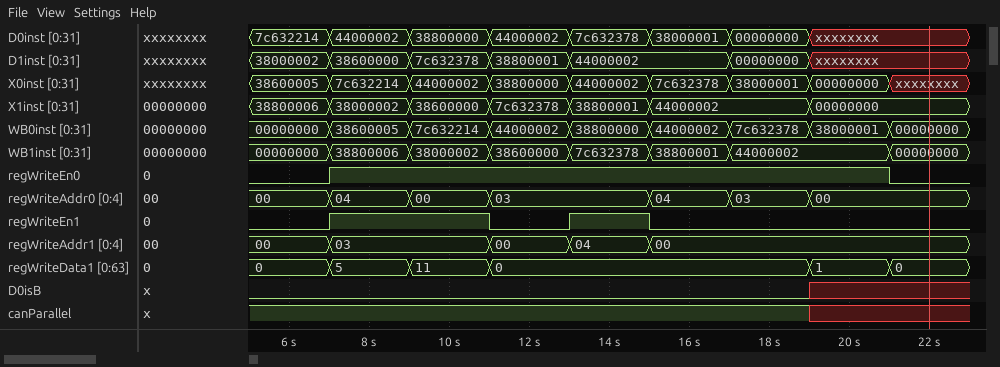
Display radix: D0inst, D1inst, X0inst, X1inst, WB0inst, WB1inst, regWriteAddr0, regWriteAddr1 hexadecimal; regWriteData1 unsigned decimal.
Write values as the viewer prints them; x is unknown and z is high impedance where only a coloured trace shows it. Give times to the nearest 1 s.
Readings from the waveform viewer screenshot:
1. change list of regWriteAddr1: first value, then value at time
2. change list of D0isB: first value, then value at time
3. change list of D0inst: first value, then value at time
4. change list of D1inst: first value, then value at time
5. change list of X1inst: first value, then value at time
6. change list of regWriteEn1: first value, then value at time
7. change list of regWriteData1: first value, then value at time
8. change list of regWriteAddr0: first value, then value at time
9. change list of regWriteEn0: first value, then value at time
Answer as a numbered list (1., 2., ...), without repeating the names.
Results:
1. 00, 03 at 7 s, 00 at 11 s, 04 at 13 s, 00 at 15 s
2. 0, x at 19 s
3. 7c632214, 44000002 at 7 s, 38800000 at 9 s, 44000002 at 11 s, 7c632378 at 13 s, 38000001 at 15 s, 00000000 at 17 s, xxxxxxxx at 19 s
4. 38000002, 38600000 at 7 s, 7c632378 at 9 s, 38800001 at 11 s, 44000002 at 13 s, 00000000 at 17 s, xxxxxxxx at 19 s
5. 38800006, 38000002 at 7 s, 38600000 at 9 s, 7c632378 at 11 s, 38800001 at 13 s, 44000002 at 15 s, 00000000 at 19 s
6. 0, 1 at 7 s, 0 at 11 s, 1 at 13 s, 0 at 15 s
7. 0, 5 at 7 s, 11 at 9 s, 0 at 11 s, 1 at 19 s, 0 at 21 s
8. 00, 04 at 7 s, 00 at 9 s, 03 at 11 s, 04 at 15 s, 03 at 17 s, 00 at 19 s
9. 0, 1 at 7 s, 0 at 21 s
